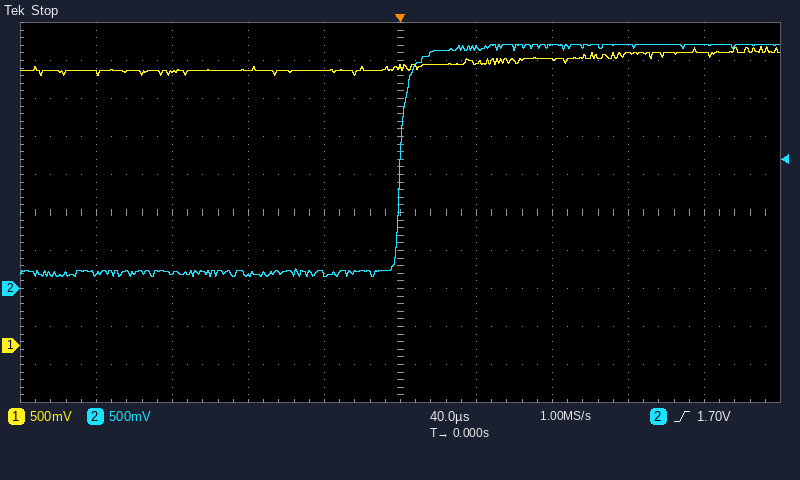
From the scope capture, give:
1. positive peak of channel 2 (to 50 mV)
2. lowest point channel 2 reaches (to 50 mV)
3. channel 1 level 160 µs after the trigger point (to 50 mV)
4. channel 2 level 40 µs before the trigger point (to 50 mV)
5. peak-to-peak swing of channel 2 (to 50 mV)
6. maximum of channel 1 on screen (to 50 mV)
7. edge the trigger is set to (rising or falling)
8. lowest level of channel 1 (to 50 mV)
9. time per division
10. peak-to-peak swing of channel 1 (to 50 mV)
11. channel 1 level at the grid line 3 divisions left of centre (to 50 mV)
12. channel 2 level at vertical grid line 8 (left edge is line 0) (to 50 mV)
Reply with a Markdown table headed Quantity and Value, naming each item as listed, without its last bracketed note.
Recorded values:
| Quantity | Value |
|---|---|
| positive peak of channel 2 | 3.20 V |
| lowest point channel 2 reaches | 150 mV |
| channel 1 level 160 µs after the trigger point | 3.85 V |
| channel 2 level 40 µs before the trigger point | 200 mV |
| peak-to-peak swing of channel 2 | 3.05 V |
| maximum of channel 1 on screen | 3.95 V |
| edge the trigger is set to | rising |
| lowest level of channel 1 | 3.55 V |
| time per division | 40 µs |
| peak-to-peak swing of channel 1 | 400 mV |
| channel 1 level at the grid line 3 divisions left of centre | 3.60 V |
| channel 2 level at vertical grid line 8 (left edge is line 0) | 3.20 V |
